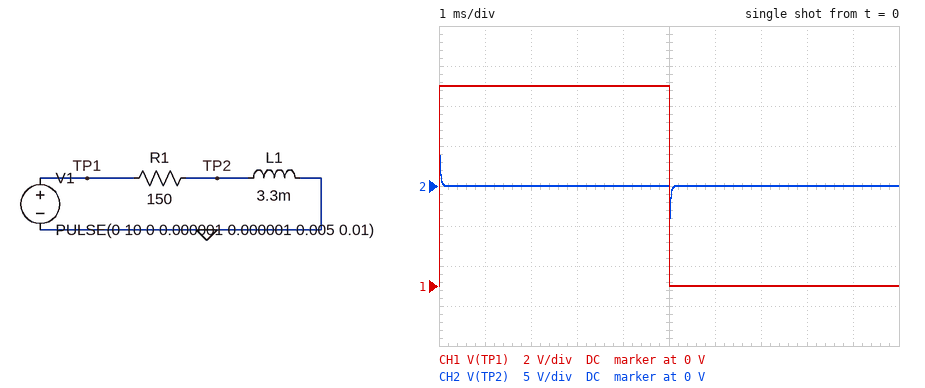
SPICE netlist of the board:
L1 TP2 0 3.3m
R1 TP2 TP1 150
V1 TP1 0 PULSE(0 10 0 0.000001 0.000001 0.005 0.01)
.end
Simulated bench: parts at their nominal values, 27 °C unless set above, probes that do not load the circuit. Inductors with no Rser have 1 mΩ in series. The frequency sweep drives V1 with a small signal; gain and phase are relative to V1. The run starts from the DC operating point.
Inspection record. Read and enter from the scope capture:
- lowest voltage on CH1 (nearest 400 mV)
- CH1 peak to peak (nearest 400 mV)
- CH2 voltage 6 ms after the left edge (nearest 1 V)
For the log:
0 V
10.0 V
0 V
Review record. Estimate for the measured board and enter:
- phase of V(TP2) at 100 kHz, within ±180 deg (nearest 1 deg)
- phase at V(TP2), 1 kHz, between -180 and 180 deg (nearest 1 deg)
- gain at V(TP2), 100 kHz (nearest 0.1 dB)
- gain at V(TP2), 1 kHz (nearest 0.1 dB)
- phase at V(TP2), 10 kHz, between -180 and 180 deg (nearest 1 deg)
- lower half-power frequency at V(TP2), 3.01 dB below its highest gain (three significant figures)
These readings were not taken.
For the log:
4 deg
82 deg
0 dB
-17.3 dB
36 deg
7.23 kHz
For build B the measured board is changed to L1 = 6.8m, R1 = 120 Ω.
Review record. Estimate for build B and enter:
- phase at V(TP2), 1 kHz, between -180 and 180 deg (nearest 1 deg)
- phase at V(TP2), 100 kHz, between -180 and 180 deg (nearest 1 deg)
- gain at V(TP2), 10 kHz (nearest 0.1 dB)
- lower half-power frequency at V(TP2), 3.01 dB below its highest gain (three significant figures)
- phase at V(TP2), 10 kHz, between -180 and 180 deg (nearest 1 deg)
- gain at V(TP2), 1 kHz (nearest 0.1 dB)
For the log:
70 deg
2 deg
-0.3 dB
2.81 kHz
16 deg
-9.5 dB
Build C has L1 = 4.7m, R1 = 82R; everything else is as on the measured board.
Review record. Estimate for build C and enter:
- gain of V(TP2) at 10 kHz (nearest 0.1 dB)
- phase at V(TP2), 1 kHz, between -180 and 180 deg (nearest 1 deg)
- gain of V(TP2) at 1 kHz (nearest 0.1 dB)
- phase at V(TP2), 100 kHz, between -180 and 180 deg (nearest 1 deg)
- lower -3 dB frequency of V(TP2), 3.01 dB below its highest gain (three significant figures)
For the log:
-0.3 dB
70 deg
-9.4 dB
2 deg
2.78 kHz
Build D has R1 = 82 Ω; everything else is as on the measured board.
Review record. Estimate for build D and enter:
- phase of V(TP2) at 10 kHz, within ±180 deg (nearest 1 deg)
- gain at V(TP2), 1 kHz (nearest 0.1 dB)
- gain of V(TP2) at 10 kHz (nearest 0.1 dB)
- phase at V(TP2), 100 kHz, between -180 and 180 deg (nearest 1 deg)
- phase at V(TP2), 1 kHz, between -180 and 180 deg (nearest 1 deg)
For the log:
22 deg
-12.2 dB
-0.6 dB
2 deg
76 deg
